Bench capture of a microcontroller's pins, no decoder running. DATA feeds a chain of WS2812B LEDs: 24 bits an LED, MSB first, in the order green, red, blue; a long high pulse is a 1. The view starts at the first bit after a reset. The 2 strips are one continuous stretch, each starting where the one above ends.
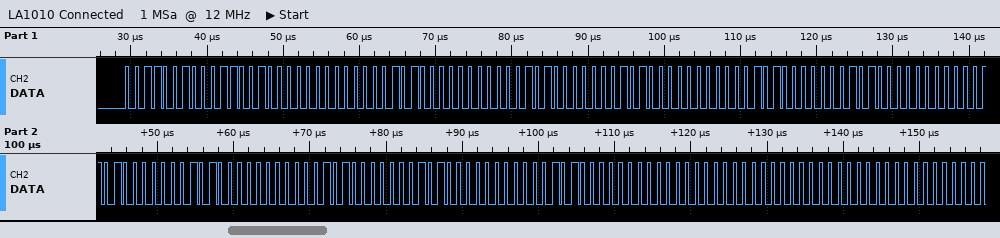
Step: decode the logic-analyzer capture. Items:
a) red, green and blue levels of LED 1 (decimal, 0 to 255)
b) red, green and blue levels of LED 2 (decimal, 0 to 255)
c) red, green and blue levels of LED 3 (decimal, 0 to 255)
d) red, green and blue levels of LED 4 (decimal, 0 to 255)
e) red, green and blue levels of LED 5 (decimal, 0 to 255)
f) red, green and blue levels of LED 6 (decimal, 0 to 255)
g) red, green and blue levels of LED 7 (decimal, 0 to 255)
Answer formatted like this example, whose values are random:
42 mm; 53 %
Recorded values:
50, 50, 0; 0, 10, 40; 0, 10, 40; 0, 10, 40; 0, 10, 40; 0, 10, 40; 0, 0, 0
